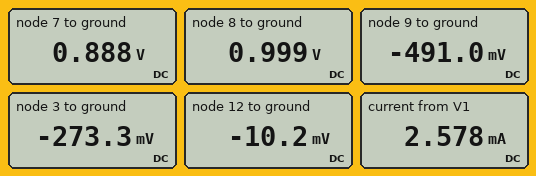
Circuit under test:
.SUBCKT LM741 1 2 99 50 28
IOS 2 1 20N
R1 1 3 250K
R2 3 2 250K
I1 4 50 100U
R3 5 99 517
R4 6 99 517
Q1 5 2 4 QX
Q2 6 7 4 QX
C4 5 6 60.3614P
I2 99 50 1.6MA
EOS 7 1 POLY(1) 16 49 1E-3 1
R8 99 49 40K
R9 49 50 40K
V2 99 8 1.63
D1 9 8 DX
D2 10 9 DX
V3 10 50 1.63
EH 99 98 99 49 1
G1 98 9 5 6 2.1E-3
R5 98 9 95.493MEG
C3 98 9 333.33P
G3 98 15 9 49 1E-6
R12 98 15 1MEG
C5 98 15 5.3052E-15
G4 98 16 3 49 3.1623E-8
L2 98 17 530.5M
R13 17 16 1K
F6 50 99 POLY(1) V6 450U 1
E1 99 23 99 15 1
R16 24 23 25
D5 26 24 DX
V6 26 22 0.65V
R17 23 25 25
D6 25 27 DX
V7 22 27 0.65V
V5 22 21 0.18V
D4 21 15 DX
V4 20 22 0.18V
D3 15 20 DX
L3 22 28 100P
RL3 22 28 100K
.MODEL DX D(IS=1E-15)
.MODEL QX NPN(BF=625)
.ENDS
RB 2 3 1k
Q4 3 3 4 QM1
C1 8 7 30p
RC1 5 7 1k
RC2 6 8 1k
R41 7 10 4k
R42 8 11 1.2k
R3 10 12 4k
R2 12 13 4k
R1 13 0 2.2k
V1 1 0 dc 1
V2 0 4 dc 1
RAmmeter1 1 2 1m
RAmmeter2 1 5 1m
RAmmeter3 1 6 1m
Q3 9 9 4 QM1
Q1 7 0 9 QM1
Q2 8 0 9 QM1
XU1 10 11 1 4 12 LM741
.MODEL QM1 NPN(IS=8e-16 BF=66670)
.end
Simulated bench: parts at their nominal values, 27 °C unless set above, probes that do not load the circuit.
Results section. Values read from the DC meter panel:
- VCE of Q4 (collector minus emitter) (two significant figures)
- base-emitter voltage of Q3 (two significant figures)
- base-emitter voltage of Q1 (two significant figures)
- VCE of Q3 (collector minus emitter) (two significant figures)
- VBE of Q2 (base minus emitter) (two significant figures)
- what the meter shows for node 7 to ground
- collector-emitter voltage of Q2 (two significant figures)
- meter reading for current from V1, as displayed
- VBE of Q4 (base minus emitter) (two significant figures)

730 mV
510 mV
490 mV
510 mV
490 mV
0.888 V
1.5 V
2.578 mA
730 mV
